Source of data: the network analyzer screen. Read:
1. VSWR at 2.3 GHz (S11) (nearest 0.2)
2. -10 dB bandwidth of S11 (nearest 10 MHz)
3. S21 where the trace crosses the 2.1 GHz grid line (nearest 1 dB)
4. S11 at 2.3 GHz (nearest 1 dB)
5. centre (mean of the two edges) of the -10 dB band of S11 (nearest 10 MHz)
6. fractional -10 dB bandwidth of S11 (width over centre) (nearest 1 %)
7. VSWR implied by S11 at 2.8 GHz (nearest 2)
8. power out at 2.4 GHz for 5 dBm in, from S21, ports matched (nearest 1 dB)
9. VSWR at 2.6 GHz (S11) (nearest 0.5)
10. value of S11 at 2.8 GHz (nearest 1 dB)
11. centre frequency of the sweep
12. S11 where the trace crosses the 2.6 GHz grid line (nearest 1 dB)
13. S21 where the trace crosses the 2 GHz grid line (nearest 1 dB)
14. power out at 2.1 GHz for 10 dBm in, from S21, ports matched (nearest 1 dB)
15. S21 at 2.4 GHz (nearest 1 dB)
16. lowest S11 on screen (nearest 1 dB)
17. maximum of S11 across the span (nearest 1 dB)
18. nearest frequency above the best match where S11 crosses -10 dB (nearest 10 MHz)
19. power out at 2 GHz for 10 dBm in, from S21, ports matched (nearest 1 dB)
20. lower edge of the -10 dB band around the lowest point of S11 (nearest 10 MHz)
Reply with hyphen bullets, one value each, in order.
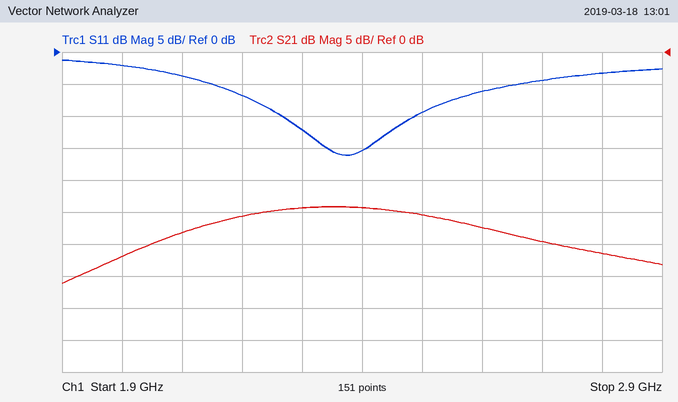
- 1.6
- 220 MHz
- -28 dB
- -12 dB
- 2.38 GHz
- 9 %
- 6
- -19 dBm
- 3.0
- -3 dB
- 2.4 GHz
- -6 dB
- -32 dB
- -18 dBm
- -24 dB
- -16 dB
- -1 dB
- 2.49 GHz
- -22 dBm
- 2.27 GHz
